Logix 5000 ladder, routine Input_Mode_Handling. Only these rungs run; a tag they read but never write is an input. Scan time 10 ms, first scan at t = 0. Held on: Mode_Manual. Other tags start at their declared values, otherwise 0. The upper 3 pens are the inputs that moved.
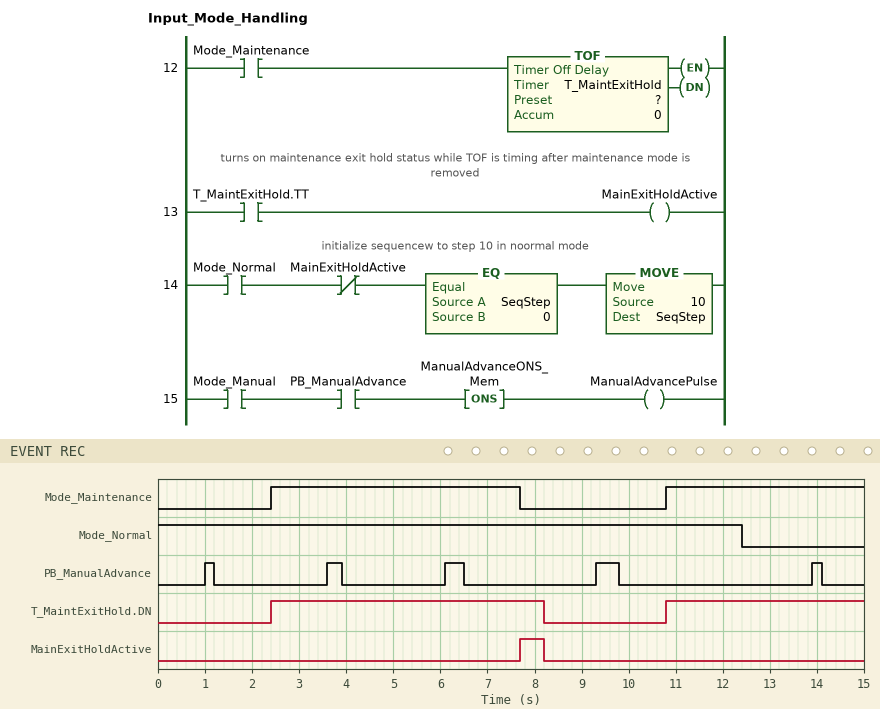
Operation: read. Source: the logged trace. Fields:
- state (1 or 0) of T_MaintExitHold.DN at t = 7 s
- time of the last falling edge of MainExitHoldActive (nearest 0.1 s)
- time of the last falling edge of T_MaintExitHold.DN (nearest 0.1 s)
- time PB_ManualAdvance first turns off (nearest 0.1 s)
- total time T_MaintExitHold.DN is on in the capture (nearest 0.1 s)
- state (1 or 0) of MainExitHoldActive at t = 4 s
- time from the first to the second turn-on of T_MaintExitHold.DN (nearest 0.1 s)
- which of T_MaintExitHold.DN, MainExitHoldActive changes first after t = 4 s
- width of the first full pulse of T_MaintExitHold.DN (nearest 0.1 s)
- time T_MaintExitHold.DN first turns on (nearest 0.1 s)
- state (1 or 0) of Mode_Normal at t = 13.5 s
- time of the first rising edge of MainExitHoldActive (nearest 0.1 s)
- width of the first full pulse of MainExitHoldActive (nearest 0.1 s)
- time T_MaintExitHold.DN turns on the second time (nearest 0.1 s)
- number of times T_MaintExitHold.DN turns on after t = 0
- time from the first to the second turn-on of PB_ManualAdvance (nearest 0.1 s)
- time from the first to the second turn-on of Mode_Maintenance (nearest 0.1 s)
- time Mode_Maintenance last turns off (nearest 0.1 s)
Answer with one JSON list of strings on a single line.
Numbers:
["1", "8.2 s", "8.2 s", "1.2 s", "10.0 s", "0", "8.4 s", "MainExitHoldActive", "5.8 s", "2.4 s", "0", "7.7 s", "0.5 s", "10.8 s", "2", "2.6 s", "8.4 s", "7.7 s"]
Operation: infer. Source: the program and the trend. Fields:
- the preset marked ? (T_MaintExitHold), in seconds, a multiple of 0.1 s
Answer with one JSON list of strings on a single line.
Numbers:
["0.5 s"]
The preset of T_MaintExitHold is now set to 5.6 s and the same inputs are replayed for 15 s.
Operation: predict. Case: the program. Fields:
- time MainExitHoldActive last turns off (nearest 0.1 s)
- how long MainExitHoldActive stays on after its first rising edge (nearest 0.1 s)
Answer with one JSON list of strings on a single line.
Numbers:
["10.8 s", "3.1 s"]
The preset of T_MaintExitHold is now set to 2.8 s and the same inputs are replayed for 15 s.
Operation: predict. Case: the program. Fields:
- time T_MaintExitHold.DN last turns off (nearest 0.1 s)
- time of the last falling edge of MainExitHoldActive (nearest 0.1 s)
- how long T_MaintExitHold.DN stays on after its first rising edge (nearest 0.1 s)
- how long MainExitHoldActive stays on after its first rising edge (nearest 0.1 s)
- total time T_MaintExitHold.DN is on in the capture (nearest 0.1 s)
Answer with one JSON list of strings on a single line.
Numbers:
["10.5 s", "10.5 s", "8.1 s", "2.8 s", "12.3 s"]
